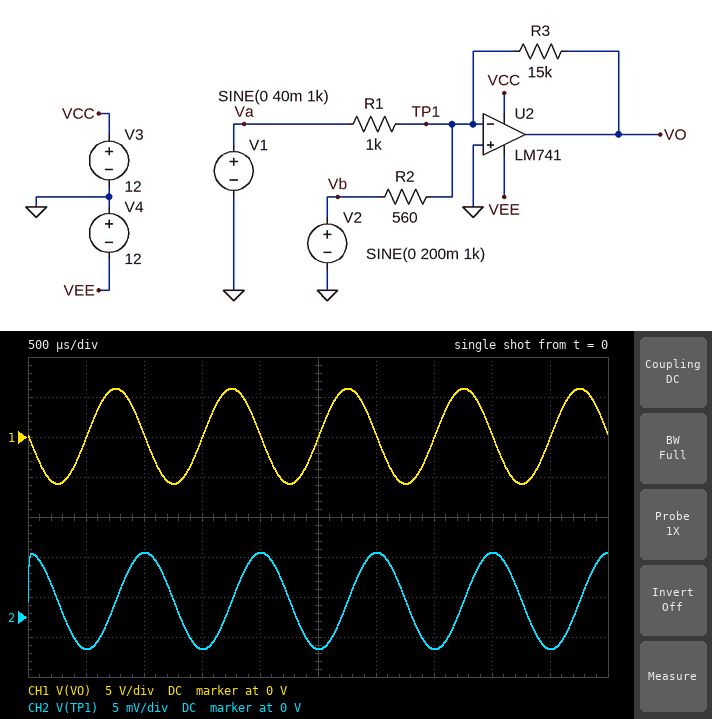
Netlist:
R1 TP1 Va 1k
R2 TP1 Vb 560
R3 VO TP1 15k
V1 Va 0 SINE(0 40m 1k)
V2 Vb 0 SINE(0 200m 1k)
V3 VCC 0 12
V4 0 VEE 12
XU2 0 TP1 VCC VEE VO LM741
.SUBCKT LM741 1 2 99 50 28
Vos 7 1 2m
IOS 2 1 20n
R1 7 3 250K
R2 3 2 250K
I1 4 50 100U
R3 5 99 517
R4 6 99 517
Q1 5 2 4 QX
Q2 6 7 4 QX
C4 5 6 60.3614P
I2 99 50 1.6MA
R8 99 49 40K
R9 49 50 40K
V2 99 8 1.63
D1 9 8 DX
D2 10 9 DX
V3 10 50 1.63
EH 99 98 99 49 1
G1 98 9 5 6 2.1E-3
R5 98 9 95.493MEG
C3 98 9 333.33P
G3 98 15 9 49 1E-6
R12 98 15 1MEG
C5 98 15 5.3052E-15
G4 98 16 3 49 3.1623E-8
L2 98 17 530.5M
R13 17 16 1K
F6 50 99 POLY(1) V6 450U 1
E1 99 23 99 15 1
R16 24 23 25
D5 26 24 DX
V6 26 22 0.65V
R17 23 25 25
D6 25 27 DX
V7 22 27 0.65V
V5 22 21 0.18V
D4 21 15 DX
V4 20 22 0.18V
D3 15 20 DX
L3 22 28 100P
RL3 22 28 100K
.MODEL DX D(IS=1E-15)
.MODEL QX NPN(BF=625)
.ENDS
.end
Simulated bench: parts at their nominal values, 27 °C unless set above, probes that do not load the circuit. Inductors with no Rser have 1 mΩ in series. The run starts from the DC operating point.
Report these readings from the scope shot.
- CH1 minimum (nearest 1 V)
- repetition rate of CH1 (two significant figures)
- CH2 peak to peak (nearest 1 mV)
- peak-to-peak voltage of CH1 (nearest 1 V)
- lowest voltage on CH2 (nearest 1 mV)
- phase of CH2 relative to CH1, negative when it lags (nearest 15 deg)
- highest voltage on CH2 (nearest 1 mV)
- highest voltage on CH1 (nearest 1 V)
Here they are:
-6 V
1.0 kHz
12 mV
12 V
-4 mV
-90 deg
8 mV
6 V
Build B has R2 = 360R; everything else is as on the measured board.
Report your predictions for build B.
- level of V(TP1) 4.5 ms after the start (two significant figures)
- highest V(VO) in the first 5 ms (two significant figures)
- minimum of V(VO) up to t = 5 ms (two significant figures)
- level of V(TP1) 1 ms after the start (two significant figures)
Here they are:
-7.1 mV
9.0 V
-8.8 V
11 mV
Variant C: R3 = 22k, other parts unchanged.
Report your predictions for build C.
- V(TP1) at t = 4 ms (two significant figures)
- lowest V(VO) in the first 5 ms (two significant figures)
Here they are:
11 mV
-8.6 V
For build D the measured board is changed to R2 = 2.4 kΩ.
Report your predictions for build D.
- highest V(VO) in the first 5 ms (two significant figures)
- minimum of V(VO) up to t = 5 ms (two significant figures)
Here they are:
1.9 V
-1.8 V
